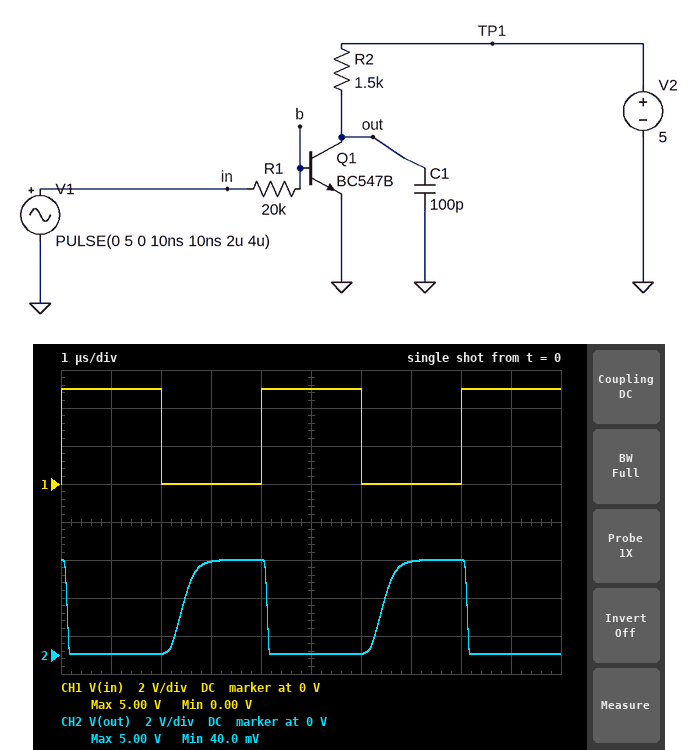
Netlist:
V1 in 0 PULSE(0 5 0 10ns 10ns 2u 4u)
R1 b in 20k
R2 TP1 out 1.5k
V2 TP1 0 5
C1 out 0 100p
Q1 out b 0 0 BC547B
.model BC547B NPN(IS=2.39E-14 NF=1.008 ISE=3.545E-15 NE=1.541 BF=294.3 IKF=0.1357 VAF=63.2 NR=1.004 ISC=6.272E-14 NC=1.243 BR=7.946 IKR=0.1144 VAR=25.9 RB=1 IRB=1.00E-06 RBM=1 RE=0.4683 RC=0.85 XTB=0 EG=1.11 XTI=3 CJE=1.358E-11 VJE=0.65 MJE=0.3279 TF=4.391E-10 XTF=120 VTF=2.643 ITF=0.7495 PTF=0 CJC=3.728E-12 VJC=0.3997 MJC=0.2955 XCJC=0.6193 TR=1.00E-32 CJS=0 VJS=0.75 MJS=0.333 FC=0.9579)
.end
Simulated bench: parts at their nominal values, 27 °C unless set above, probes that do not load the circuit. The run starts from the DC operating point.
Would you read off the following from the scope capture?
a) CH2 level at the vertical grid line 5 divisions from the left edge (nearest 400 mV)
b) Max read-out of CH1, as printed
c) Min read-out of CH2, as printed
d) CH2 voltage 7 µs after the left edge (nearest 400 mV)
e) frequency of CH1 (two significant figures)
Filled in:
0 V
5.00 V
40.0 mV
4.8 V
250 kHz
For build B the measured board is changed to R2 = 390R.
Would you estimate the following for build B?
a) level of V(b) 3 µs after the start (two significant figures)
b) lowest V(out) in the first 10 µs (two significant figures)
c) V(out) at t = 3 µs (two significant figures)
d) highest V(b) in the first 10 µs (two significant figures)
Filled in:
210 mV
89 mV
5.0 V
720 mV
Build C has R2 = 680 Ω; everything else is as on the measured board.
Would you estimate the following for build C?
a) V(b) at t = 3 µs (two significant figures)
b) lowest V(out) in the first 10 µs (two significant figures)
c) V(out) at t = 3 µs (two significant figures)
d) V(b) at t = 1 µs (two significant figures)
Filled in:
230 mV
66 mV
5.0 V
700 mV
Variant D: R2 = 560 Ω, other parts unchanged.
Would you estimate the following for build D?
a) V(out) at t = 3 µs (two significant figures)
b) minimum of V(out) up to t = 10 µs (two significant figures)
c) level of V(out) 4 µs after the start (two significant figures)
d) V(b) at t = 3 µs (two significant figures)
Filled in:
5.0 V
73 mV
5.0 V
220 mV
